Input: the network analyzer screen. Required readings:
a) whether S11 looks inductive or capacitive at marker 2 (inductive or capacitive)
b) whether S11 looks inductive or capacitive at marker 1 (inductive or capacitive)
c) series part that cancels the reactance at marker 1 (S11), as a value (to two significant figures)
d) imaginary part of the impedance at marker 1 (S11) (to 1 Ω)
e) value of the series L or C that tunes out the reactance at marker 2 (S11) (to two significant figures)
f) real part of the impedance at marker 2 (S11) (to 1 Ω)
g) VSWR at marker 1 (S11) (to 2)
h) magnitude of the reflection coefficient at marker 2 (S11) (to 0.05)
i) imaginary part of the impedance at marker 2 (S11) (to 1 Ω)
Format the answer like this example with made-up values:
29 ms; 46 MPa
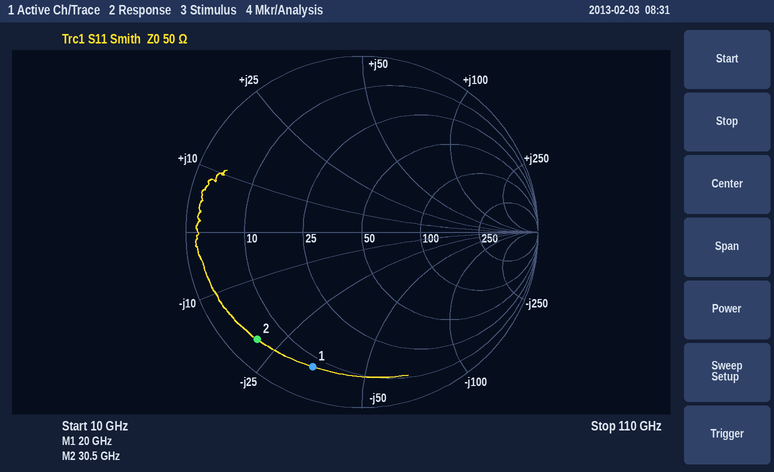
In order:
capacitive; capacitive; 270 pH; -34 Ω; 110 pH; 5 Ω; 10; 0.85; -21 Ω
